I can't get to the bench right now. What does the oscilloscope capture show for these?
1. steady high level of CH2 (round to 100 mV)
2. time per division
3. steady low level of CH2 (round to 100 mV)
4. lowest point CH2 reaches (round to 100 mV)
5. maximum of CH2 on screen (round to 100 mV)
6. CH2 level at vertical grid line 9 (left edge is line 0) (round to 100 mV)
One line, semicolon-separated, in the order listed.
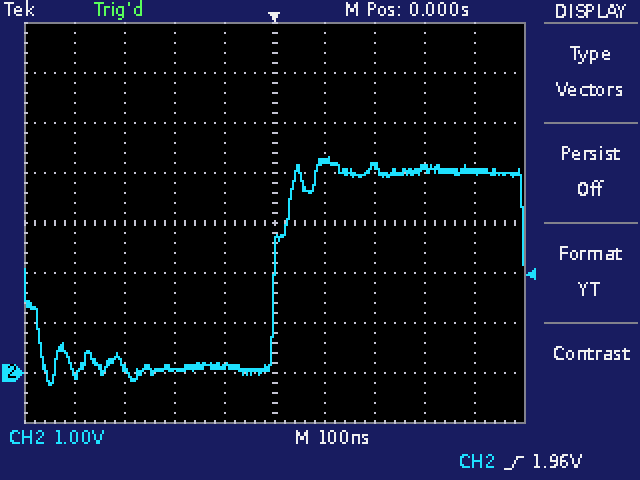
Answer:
4.0 V; 100 ns; 100 mV; -200 mV; 4.3 V; 4.0 V
